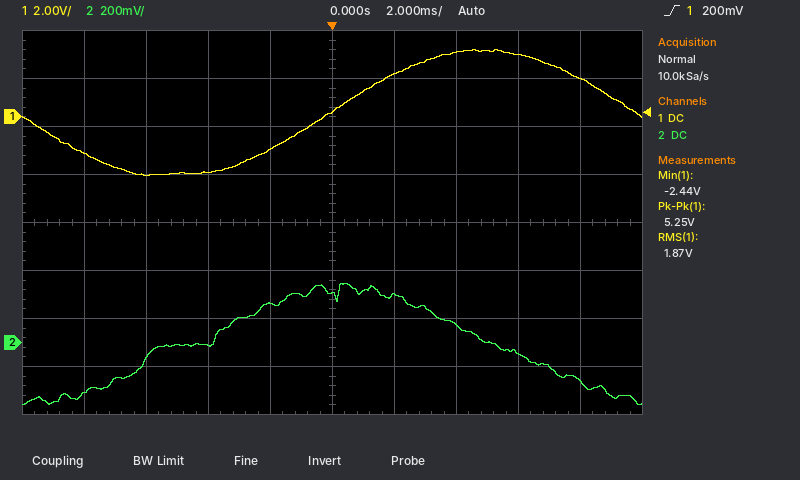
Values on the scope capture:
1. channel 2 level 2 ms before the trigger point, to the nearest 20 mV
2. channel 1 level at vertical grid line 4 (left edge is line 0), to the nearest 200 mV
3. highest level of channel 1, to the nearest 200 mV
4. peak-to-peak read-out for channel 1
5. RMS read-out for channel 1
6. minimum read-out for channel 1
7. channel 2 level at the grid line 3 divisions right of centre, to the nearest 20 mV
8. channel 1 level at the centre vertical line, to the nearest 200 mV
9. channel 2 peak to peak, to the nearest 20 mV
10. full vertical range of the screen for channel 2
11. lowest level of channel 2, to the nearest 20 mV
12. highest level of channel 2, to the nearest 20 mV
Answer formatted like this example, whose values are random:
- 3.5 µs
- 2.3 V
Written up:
- 160 mV
- -1.4 V
- 2.8 V
- 5.25 V
- 1.87 V
- -2.44 V
- -40 mV
- 200 mV
- 500 mV
- 1.6 V
- -260 mV
- 240 mV
